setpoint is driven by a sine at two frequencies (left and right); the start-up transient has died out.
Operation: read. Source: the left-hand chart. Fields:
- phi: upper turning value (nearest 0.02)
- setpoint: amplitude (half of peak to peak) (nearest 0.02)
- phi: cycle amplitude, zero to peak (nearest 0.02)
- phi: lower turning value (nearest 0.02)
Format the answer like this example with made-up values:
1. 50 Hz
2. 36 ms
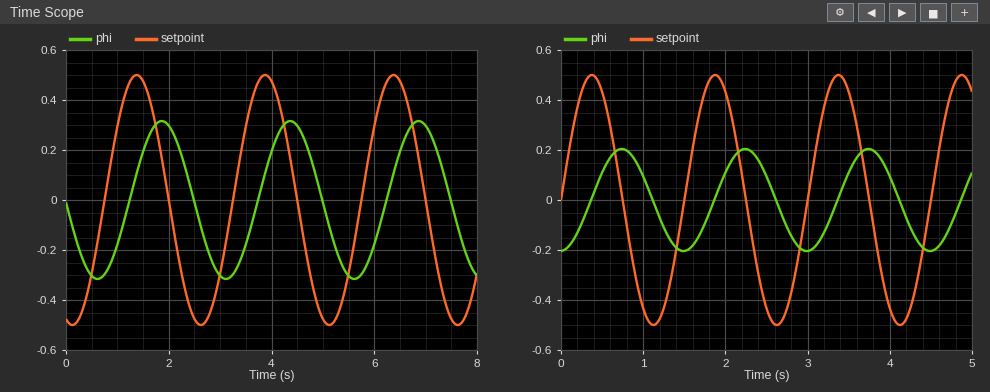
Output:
1. 0.32
2. 0.50
3. 0.32
4. -0.32
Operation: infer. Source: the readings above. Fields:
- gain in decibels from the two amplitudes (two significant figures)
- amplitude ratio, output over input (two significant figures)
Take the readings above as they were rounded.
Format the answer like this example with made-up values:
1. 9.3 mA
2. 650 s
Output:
1. -3.9 dB
2. 0.64
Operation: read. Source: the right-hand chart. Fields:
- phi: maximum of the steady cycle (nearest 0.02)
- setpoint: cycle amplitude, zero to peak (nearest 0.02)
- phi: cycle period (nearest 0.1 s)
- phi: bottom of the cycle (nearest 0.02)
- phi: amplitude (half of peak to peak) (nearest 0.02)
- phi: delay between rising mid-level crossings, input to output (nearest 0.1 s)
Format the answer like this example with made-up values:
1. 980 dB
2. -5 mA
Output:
1. 0.20
2. 0.50
3. 1.5 s
4. -0.20
5. 0.20
6. 0.4 s
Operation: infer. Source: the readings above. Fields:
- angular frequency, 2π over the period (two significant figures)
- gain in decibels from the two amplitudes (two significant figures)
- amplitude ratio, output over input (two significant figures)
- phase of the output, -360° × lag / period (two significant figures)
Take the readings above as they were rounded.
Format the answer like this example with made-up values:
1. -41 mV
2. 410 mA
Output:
1. 4.2 rad/s
2. -8.0 dB
3. 0.40
4. -96°
